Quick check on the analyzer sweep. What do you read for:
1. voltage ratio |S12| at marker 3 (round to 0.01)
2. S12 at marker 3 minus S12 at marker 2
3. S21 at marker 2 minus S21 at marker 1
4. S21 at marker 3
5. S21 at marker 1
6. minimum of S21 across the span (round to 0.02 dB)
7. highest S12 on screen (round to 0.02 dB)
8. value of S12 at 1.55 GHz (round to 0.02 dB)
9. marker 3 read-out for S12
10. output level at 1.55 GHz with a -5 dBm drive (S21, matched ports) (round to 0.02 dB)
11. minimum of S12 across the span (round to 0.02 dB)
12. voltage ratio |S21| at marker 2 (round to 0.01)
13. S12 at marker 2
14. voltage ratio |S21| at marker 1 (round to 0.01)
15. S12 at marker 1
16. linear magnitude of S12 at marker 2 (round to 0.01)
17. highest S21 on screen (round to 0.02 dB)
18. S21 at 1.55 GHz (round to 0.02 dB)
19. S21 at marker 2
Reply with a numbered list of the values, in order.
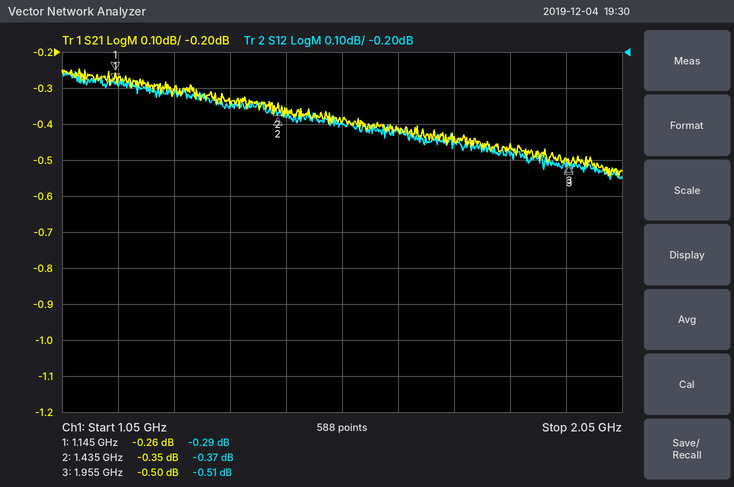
1. 0.94
2. -0.14 dB
3. -0.09 dB
4. -0.50 dB
5. -0.26 dB
6. -0.54 dB
7. -0.26 dB
8. -0.40 dB
9. -0.51 dB
10. -5.40 dBm
11. -0.56 dB
12. 0.96
13. -0.37 dB
14. 0.97
15. -0.29 dB
16. 0.96
17. -0.24 dB
18. -0.40 dB
19. -0.35 dB
